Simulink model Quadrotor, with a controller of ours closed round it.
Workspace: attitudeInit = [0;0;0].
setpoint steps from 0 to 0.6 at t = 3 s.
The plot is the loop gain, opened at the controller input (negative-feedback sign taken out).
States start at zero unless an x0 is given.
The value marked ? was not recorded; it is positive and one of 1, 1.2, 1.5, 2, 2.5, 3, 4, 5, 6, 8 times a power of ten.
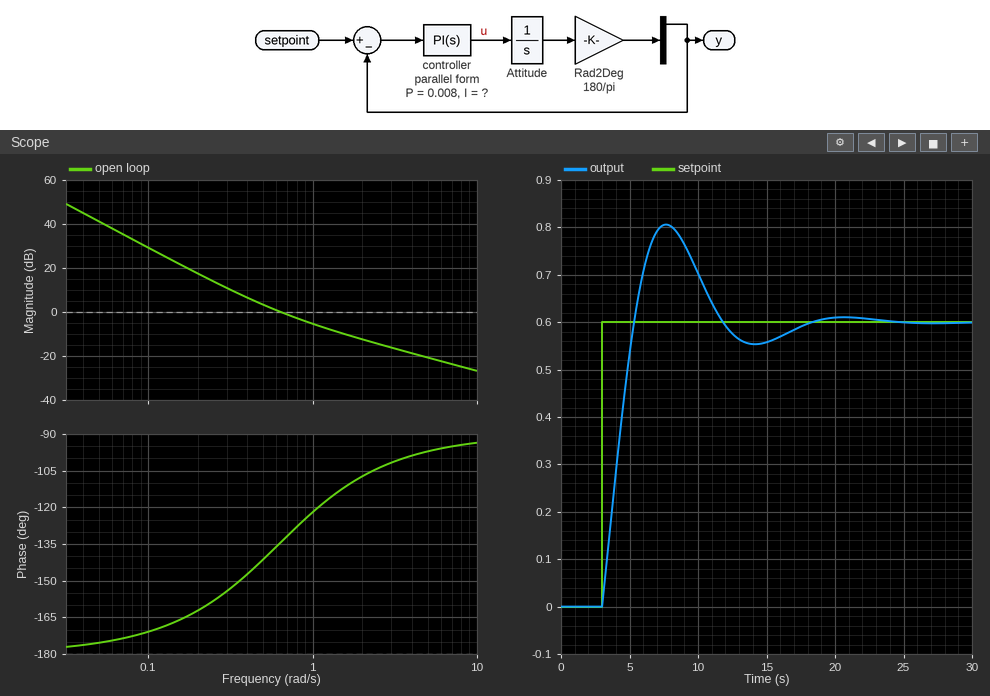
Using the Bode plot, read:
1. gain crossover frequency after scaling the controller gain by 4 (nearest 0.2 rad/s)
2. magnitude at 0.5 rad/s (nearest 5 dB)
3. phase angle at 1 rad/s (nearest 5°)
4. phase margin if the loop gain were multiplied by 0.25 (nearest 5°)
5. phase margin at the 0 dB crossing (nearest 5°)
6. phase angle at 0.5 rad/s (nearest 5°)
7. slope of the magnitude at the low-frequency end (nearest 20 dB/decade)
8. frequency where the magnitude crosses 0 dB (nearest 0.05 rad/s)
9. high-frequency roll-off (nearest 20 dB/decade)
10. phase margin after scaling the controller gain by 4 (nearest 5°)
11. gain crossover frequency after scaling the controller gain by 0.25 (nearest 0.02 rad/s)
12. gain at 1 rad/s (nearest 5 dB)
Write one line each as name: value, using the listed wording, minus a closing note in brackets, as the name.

gain crossover frequency after scaling the controller gain by 4: 2.0 rad/s
magnitude at 0.5 rad/s: 5 dB
phase angle at 1 rad/s: -120°
phase margin if the loop gain were multiplied by 0.25: 25°
phase margin at the 0 dB crossing: 45°
phase angle at 0.5 rad/s: -140°
slope of the magnitude at the low-frequency end: -40 dB/decade
frequency where the magnitude crosses 0 dB: 0.65 rad/s
high-frequency roll-off: -20 dB/decade
phase margin after scaling the controller gain by 4: 70°
gain crossover frequency after scaling the controller gain by 0.25: 0.28 rad/s
gain at 1 rad/s: -5 dB
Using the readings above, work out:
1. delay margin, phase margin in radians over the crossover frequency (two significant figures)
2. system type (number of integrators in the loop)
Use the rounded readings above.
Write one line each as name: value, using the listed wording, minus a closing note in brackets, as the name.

delay margin, phase margin in radians over the crossover frequency: 1.2 s
system type: 2
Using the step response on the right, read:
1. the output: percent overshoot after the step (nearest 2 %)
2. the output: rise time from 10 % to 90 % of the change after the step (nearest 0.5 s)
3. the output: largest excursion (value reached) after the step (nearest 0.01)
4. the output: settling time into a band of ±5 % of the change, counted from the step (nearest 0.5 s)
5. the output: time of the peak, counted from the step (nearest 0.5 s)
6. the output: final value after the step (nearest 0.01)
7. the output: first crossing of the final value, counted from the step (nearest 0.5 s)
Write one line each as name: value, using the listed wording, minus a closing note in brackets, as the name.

the output: percent overshoot after the step: 34 %
the output: rise time from 10 % to 90 % of the change after the step: 2.0 s
the output: largest excursion (value reached) after the step: 0.81
the output: settling time into a band of ±5 % of the change, counted from the step: 13.0 s
the output: time of the peak, counted from the step: 4.5 s
the output: final value after the step: 0.60
the output: first crossing of the final value, counted from the step: 2.5 s
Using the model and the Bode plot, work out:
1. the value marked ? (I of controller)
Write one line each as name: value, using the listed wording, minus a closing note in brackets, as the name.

the value marked ?: 0.005
